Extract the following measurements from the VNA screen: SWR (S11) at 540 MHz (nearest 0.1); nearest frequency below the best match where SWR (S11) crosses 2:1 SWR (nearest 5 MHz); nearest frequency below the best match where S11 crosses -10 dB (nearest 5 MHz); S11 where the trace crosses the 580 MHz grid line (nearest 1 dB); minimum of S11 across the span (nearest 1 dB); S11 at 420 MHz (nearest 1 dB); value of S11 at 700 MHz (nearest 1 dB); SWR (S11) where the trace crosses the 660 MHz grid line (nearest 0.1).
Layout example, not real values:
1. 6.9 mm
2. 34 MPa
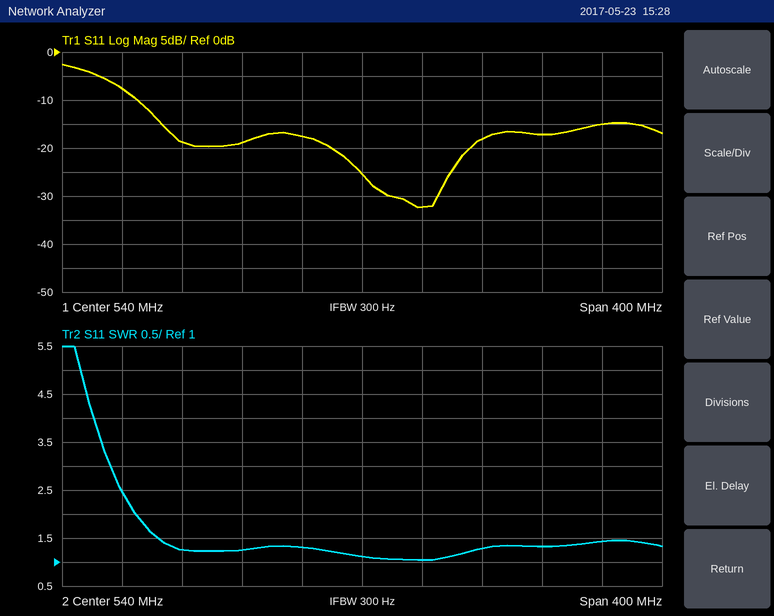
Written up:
1. 1.1
2. 390 MHz
3. 390 MHz
4. -32 dB
5. -32 dB
6. -19 dB
7. -15 dB
8. 1.3
